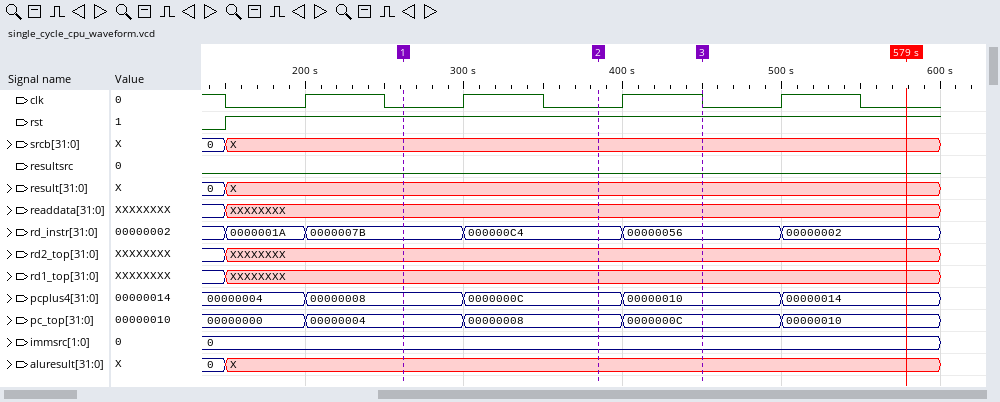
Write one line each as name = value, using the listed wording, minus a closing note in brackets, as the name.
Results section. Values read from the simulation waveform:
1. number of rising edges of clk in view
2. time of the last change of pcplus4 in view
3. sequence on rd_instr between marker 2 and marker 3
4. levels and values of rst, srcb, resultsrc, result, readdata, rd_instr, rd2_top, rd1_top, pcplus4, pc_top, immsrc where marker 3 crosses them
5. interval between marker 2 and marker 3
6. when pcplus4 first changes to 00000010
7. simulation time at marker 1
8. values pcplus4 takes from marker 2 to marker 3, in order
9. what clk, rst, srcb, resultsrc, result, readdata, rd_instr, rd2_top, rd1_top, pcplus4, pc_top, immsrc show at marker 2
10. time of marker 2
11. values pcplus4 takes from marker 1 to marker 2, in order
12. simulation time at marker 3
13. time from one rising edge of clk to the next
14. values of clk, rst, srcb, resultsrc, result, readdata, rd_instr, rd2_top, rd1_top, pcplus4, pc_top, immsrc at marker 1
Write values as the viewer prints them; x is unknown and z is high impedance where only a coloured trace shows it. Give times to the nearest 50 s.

number of rising edges of clk in view = 4
time of the last change of pcplus4 in view = 500 s
sequence on rd_instr between marker 2 and marker 3 = 000000C4, 00000056
levels and values of rst, srcb, resultsrc, result, readdata, rd_instr, rd2_top, rd1_top, pcplus4, pc_top, immsrc where marker 3 crosses them = rst=1, srcb=X, resultsrc=0, result=X, readdata=XXXXXXXX, rd_instr=00000056, rd2_top=XXXXXXXX, rd1_top=XXXXXXXX, pcplus4=00000010, pc_top=0000000C, immsrc=0
interval between marker 2 and marker 3 = 50 s
when pcplus4 first changes to 00000010 = 400 s
simulation time at marker 1 = 250 s
values pcplus4 takes from marker 2 to marker 3, in order = 0000000C, 00000010
what clk, rst, srcb, resultsrc, result, readdata, rd_instr, rd2_top, rd1_top, pcplus4, pc_top, immsrc show at marker 2 = clk=0, rst=1, srcb=X, resultsrc=0, result=X, readdata=XXXXXXXX, rd_instr=000000C4, rd2_top=XXXXXXXX, rd1_top=XXXXXXXX, pcplus4=0000000C, pc_top=00000008, immsrc=0
time of marker 2 = 400 s
values pcplus4 takes from marker 1 to marker 2, in order = 00000008, 0000000C
simulation time at marker 3 = 450 s
time from one rising edge of clk to the next = 100 s
values of clk, rst, srcb, resultsrc, result, readdata, rd_instr, rd2_top, rd1_top, pcplus4, pc_top, immsrc at marker 1 = clk=0, rst=1, srcb=X, resultsrc=0, result=X, readdata=XXXXXXXX, rd_instr=0000007B, rd2_top=XXXXXXXX, rd1_top=XXXXXXXX, pcplus4=00000008, pc_top=00000004, immsrc=0
